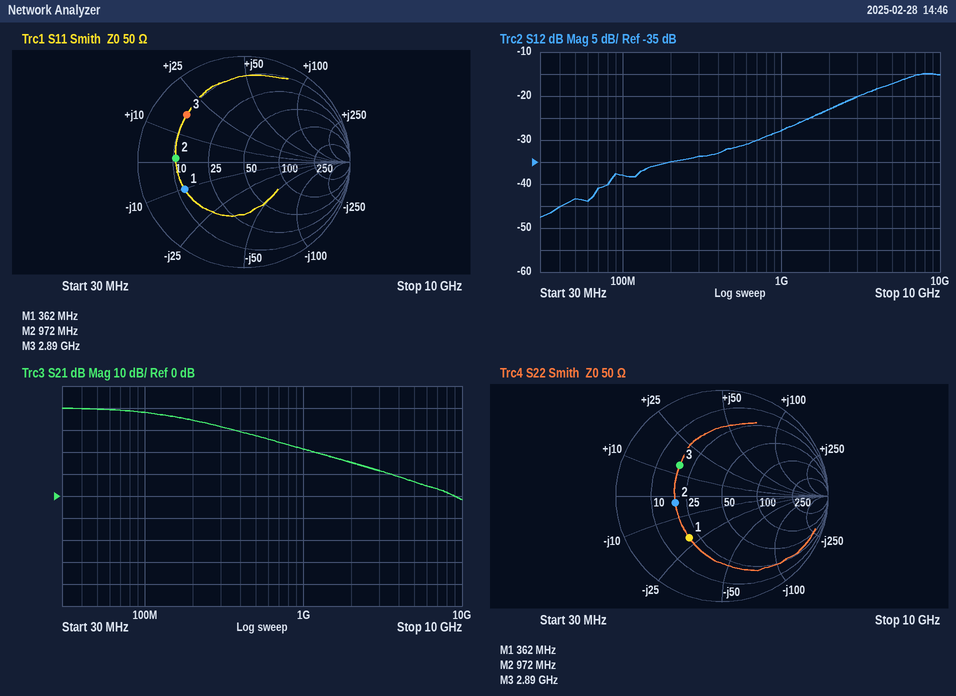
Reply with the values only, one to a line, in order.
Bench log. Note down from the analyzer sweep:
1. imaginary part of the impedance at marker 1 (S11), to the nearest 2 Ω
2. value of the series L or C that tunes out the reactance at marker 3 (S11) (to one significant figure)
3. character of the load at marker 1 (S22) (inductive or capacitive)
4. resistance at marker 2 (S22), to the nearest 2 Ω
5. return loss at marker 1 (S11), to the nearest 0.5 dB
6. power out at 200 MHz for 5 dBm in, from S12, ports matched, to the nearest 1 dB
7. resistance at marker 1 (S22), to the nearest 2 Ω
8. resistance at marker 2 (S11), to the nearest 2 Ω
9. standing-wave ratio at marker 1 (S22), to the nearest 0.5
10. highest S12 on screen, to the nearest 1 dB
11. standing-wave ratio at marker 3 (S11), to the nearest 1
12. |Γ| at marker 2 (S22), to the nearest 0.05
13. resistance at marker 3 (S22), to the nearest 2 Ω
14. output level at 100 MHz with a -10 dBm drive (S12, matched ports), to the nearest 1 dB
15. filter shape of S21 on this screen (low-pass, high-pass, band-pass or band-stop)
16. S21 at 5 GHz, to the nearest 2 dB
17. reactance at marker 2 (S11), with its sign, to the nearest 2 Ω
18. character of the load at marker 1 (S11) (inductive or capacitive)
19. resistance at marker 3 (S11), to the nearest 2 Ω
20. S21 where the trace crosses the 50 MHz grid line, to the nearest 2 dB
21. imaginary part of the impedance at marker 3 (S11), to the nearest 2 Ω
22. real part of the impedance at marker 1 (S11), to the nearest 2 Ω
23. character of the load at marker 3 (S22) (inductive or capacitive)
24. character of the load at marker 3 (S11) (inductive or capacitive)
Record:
-10 Ω
3 pF
capacitive
20 Ω
4.0 dB
-30 dBm
20 Ω
10 Ω
3.0
-15 dB
6
0.45
18 Ω
-48 dBm
low-pass
6 dB
+2 Ω
capacitive
10 Ω
40 dB
+18 Ω
12 Ω
inductive
inductive
